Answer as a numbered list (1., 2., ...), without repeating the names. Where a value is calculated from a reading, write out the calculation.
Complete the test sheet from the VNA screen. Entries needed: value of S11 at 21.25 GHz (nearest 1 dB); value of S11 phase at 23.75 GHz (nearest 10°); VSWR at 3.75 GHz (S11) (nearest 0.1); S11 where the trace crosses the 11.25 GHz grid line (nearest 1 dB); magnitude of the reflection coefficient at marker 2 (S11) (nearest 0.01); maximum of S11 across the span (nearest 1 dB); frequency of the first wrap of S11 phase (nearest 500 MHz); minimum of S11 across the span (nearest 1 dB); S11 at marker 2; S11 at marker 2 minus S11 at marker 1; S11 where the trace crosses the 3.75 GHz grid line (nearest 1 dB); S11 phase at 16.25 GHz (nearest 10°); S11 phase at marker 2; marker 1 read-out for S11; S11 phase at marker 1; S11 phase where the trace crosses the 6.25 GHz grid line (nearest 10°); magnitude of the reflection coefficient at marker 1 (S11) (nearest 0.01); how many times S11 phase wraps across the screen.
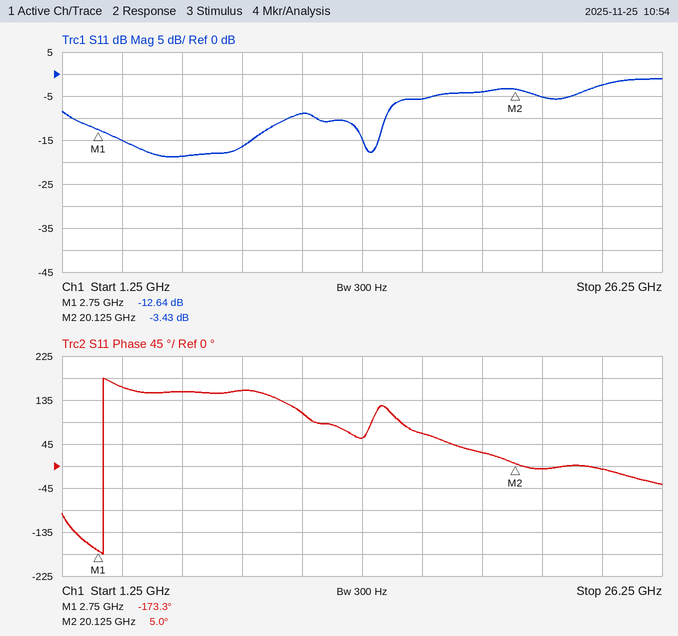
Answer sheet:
1. -5 dB
2. -10°
3. |Γ| = 10^(-15/20) = 0.1778; VSWR = (1 + 0.1778)/(1 − 0.1778) ≈ 1.4
4. -9 dB
5. 10^(-3.43/20) ≈ 0.67
6. -1 dB
7. 3.0 GHz
8. -19 dB
9. -3.43 dB
10. -3.43 − (-12.64) = 9.21 dB
11. -15 dB
12. 70°
13. 5.0°
14. -12.64 dB
15. -173.3°
16. 150°
17. 10^(-12.64/20) ≈ 0.23
18. 1
